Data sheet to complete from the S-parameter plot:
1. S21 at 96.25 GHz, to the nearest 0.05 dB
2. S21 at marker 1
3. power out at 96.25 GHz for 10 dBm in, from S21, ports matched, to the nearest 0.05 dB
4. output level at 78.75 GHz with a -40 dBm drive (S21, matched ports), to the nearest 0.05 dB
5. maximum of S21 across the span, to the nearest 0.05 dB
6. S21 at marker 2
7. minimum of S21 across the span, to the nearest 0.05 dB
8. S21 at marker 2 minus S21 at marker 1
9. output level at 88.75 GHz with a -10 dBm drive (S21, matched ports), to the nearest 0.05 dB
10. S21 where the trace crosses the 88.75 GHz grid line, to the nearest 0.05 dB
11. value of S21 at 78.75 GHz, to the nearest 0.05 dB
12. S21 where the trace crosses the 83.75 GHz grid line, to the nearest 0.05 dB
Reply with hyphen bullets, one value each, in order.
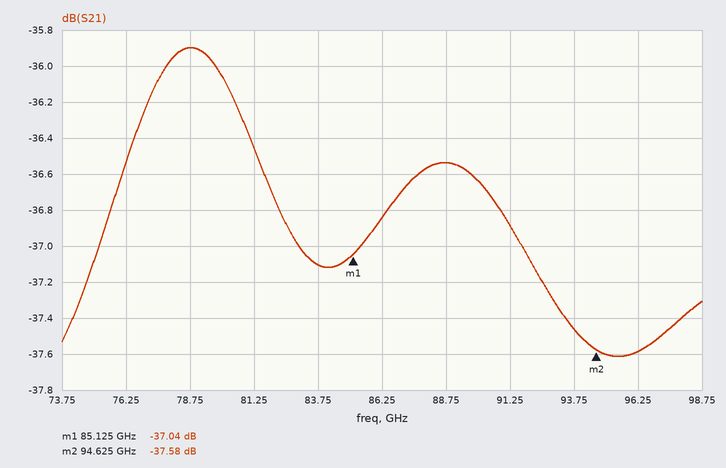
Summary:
- -37.60 dB
- -37.04 dB
- -27.60 dBm
- -75.90 dBm
- -35.90 dB
- -37.58 dB
- -37.60 dB
- -0.54 dB
- -46.55 dBm
- -36.55 dB
- -35.90 dB
- -37.10 dB
